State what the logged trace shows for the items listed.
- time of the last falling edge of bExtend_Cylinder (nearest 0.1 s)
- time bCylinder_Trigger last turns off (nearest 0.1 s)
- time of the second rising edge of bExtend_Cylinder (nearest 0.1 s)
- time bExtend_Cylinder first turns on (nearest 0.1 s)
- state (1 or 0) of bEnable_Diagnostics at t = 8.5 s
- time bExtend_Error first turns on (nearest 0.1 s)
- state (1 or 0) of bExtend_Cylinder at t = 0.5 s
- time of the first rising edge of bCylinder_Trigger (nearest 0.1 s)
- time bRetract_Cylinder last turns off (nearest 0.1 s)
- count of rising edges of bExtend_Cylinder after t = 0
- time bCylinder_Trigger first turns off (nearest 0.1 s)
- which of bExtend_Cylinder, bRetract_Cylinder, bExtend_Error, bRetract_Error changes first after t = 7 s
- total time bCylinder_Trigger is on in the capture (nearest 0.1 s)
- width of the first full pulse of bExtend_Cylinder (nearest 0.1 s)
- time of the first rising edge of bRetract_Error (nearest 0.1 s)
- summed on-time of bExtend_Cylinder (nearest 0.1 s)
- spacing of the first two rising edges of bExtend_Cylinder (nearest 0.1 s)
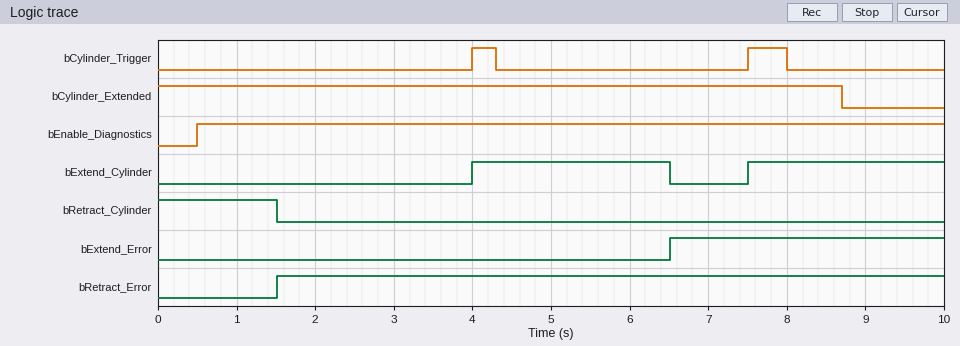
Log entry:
6.5 s
8.0 s
7.5 s
4.0 s
1
6.5 s
0
4.0 s
1.5 s
2
4.3 s
bExtend_Cylinder
0.8 s
2.5 s
1.5 s
5.0 s
3.5 s
